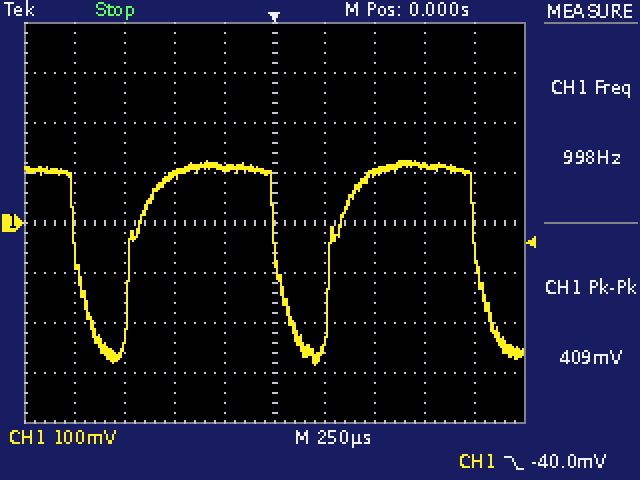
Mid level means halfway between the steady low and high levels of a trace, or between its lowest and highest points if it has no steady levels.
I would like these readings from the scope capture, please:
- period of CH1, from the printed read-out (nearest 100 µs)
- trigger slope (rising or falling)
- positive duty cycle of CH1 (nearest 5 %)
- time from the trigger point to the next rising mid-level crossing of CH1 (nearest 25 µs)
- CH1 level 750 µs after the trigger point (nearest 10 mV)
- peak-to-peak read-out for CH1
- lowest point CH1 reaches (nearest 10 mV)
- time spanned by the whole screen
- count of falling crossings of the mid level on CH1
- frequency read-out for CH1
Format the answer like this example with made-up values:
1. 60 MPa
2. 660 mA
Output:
1. 1.0 ms
2. falling
3. 75 %
4. 275 µs
5. 110 mV
6. 409 mV
7. -280 mV
8. 2.5 ms
9. 3
10. 998 Hz
